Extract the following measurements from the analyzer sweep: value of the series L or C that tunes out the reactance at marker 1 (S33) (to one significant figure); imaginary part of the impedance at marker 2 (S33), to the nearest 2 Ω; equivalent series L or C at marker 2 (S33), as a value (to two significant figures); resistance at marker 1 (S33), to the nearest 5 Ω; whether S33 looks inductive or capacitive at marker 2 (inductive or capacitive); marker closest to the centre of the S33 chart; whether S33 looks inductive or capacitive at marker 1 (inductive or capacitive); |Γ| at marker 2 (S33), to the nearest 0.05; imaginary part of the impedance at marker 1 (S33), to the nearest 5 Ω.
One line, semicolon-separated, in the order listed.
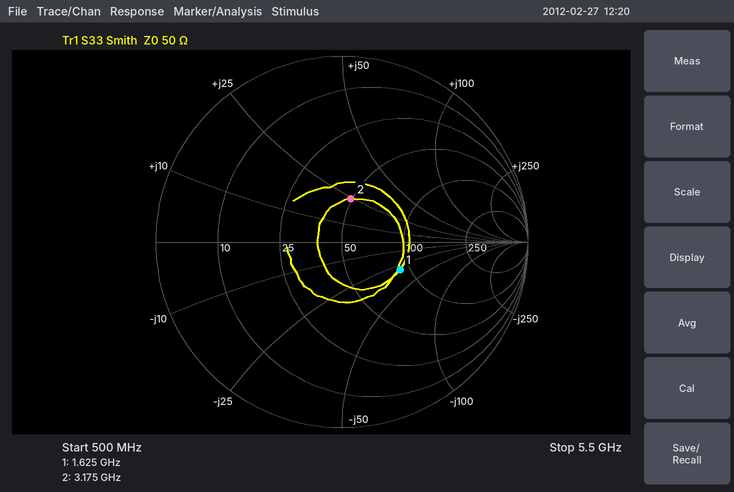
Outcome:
3 nH; +24 Ω; 1.2 nH; 90 Ω; inductive; marker 2; capacitive; 0.25; -30 Ω
